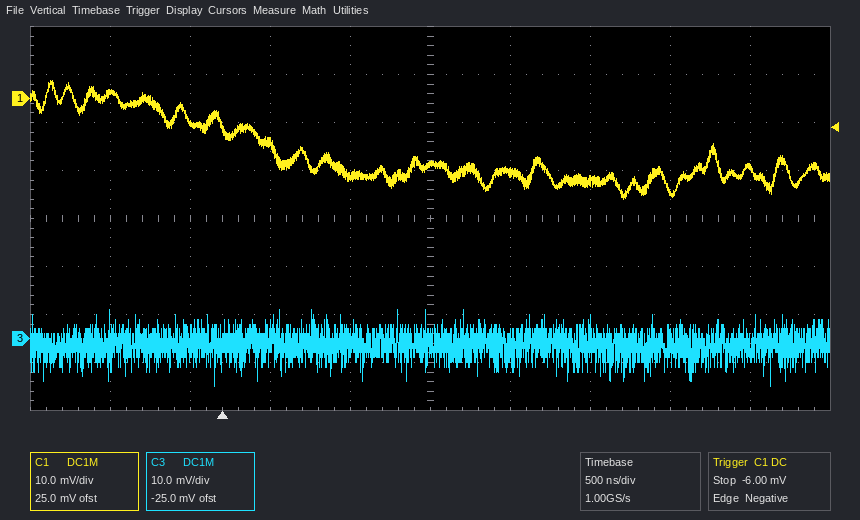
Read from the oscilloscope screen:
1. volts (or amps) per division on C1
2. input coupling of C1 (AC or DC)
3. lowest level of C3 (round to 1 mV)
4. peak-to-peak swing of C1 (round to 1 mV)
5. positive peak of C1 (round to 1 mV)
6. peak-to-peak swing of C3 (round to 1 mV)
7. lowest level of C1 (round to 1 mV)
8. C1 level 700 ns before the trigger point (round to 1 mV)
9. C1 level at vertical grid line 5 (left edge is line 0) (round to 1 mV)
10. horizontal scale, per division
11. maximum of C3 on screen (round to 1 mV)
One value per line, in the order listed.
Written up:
10 mV
DC
-10 mV
25 mV
4 mV
16 mV
-21 mV
1 mV
-14 mV
500 ns
6 mV
